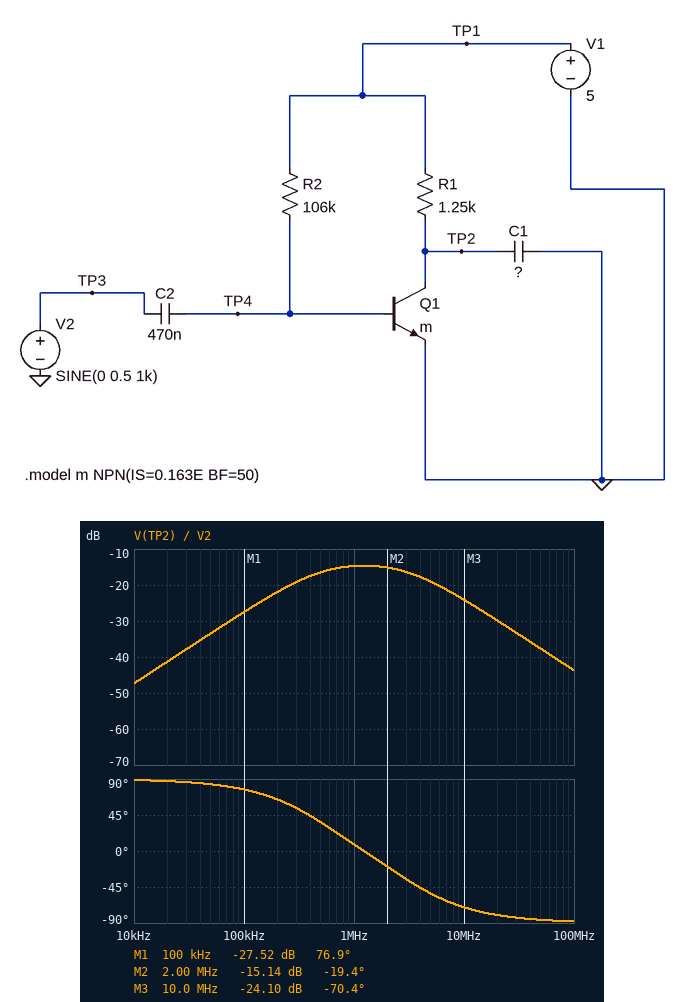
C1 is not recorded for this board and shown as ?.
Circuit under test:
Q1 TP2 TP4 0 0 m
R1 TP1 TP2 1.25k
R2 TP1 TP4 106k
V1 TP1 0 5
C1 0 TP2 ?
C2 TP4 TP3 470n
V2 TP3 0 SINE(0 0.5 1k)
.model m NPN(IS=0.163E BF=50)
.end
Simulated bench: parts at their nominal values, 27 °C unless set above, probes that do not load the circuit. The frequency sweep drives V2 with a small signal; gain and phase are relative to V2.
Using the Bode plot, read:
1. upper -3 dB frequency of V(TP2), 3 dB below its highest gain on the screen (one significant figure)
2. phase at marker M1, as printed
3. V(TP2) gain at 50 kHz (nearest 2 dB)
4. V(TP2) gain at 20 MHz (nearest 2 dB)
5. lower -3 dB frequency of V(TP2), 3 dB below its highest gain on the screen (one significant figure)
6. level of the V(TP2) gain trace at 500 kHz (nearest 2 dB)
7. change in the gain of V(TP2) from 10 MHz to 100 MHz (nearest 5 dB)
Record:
4 MHz
76.9 deg
-34 dB
-30 dB
400 kHz
-16 dB
-20 dB
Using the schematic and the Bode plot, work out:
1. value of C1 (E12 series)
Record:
1.5 µF
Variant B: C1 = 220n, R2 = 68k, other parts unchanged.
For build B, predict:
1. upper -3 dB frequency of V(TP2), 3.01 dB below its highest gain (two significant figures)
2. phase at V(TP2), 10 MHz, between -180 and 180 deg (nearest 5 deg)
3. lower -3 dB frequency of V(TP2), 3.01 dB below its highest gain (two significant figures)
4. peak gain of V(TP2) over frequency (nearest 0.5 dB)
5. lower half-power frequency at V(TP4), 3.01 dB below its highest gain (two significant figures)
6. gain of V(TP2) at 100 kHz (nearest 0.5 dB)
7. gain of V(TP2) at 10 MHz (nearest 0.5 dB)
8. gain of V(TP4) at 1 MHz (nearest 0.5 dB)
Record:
12 MHz
-40 deg
850 kHz
-8.0 dB
1.3 MHz
-27.5 dB
-10.0 dB
-4.0 dB
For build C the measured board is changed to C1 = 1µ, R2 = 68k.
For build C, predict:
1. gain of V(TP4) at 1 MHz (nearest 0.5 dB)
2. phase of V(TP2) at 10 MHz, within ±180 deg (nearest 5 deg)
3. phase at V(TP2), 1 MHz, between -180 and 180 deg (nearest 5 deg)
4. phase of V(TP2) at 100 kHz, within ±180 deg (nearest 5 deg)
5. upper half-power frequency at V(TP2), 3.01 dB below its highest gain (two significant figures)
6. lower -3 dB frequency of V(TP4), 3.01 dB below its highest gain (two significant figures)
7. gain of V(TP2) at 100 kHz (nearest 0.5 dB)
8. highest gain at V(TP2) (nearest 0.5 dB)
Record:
-6.0 dB
-65 deg
15 deg
80 deg
4.7 MHz
2.4 MHz
-27.5 dB
-12.5 dB
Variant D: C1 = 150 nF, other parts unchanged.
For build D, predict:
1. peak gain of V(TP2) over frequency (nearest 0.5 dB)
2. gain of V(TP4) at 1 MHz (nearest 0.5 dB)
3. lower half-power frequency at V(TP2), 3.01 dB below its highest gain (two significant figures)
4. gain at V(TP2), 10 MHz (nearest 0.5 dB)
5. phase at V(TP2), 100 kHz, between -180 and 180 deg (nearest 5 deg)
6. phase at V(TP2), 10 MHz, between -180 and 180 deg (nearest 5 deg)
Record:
-7.5 dB
-4.0 dB
920 kHz
-8.5 dB
85 deg
-30 deg
